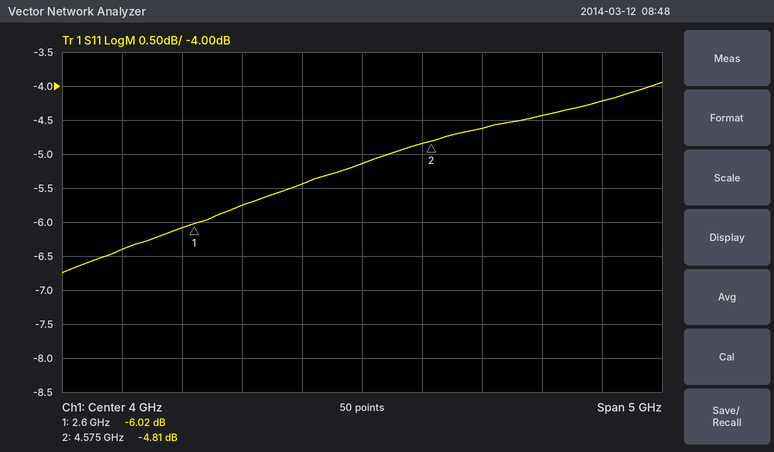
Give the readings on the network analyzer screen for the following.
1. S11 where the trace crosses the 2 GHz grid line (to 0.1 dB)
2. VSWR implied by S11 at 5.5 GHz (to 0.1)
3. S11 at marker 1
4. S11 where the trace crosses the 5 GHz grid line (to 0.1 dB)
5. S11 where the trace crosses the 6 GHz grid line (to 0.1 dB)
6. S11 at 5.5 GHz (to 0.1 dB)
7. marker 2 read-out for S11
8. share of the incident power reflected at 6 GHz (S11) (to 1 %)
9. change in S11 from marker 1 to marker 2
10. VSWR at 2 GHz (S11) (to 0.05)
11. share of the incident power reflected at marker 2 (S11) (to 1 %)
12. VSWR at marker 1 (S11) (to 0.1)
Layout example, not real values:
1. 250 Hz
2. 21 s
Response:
1. -6.4 dB
2. 4.0
3. -6.02 dB
4. -4.6 dB
5. -4.2 dB
6. -4.4 dB
7. -4.81 dB
8. 38 %
9. 1.21 dB
10. 2.85
11. 33 %
12. 3.0
